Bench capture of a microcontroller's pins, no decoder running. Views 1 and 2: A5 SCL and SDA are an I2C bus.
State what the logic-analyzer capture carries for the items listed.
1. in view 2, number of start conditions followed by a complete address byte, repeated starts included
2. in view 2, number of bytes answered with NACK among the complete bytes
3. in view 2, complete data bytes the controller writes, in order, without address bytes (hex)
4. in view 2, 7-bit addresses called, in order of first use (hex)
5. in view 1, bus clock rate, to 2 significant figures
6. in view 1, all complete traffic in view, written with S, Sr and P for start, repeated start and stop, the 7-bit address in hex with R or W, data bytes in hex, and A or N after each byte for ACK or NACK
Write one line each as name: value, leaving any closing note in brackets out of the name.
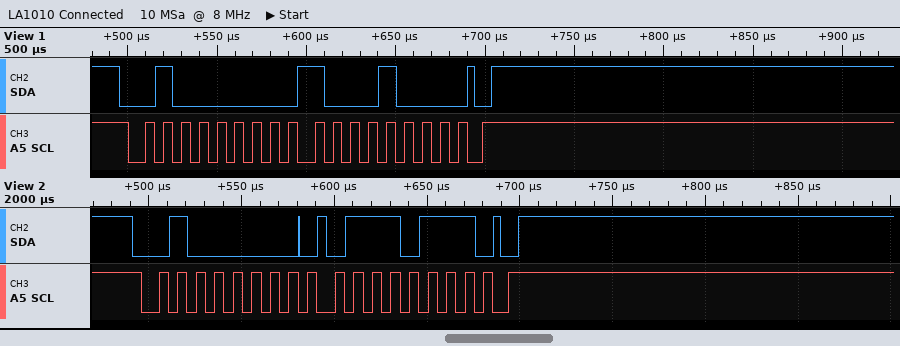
in view 2, number of start conditions followed by a complete address byte, repeated starts included: 1
in view 2, number of bytes answered with NACK among the complete bytes: 0
in view 2, complete data bytes the controller writes, in order, without address bytes: 77
in view 2, 7-bit addresses called, in order of first use: 0x20
in view 1, bus clock rate, to 2 significant figures: 100 kHz
in view 1, all complete traffic in view, written with S, Sr and P for start, repeated start and stop, the 7-bit address in hex with R or W, data bytes in hex, and A or N after each byte for ACK or NACK: S 20W A 88 A P
